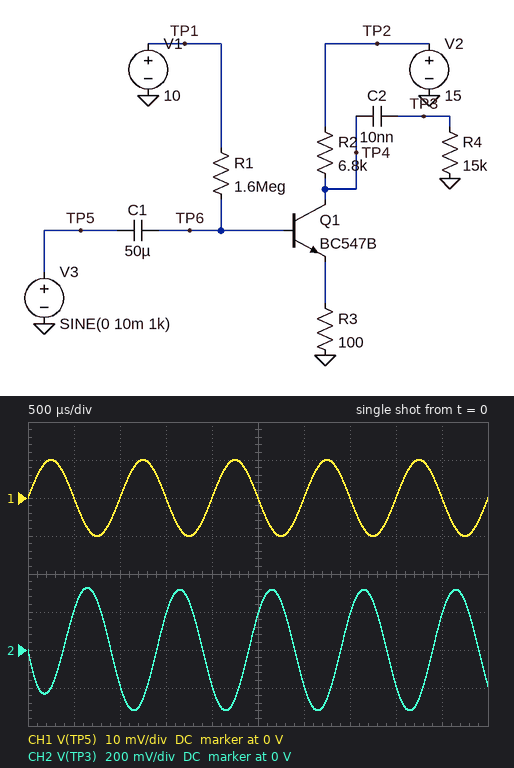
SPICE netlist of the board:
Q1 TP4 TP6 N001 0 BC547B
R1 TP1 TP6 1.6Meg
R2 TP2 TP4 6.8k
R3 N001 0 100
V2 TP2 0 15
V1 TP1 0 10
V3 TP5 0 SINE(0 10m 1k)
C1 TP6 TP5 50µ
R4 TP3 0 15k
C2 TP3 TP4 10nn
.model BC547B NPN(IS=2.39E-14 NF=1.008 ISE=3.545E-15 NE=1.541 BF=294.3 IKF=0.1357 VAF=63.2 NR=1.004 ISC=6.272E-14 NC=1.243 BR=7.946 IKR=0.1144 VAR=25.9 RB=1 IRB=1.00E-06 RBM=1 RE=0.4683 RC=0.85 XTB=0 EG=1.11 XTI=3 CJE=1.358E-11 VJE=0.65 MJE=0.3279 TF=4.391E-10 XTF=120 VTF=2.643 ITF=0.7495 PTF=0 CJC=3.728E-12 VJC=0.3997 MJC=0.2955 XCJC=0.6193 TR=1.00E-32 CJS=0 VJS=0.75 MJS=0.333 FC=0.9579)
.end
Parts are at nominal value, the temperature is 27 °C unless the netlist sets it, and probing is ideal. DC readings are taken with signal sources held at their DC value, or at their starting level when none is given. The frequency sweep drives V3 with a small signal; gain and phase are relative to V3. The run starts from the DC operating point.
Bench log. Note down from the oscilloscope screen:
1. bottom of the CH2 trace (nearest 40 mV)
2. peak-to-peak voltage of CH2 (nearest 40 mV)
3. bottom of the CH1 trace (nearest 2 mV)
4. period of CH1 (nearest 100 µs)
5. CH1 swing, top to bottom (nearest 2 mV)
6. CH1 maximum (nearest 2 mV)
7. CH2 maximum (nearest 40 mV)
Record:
-320 mV
640 mV
-10 mV
1.0 ms
20 mV
10 mV
320 mV
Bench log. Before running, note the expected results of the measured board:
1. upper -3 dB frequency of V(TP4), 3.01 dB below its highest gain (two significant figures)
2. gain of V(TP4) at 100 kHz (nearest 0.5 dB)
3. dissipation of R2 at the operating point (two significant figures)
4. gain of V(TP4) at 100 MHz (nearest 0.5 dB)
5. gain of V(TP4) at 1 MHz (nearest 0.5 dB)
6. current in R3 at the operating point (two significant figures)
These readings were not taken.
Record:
3.7 kHz
32.0 dB
19 mW
15.5 dB
32.0 dB
1.7 mA
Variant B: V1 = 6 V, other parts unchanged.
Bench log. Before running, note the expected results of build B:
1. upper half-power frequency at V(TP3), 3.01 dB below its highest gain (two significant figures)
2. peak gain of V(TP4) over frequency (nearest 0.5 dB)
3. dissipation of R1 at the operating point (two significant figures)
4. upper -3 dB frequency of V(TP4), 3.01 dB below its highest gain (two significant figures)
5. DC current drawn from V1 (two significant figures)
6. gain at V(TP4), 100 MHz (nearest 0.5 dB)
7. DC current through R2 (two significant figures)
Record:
21 MHz
34.5 dB
17 µW
3.6 kHz
3.3 µA
16.5 dB
1.0 mA
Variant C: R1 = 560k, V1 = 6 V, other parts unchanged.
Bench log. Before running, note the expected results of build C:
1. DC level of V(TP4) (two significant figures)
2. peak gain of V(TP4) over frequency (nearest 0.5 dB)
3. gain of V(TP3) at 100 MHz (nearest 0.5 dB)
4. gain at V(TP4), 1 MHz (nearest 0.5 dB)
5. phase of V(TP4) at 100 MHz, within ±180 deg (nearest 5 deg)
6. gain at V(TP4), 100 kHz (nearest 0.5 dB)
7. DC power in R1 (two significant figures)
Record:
370 mV
31.5 dB
2.0 dB
28.0 dB
15 deg
29.5 dB
47 µW
